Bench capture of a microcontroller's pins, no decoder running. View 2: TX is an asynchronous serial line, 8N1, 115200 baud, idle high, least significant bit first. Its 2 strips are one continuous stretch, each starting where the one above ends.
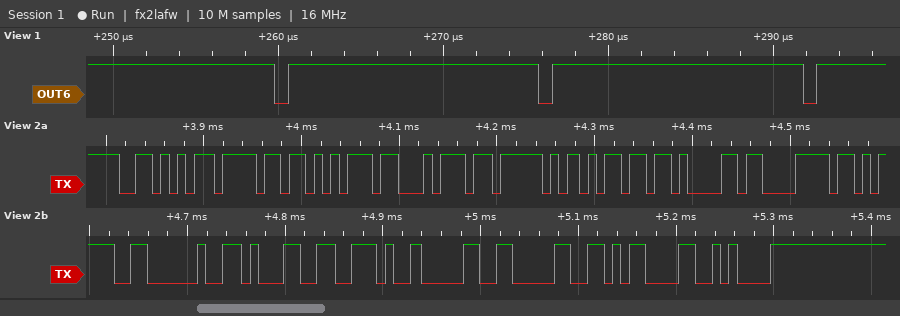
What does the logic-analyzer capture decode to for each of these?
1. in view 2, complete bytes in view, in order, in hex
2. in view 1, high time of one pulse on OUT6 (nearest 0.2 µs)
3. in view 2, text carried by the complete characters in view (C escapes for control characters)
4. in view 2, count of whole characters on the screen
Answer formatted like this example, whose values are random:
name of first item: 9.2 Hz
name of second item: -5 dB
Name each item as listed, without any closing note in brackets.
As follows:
in view 2, complete bytes in view, in order, in hex: 56 6F 75 74 5F 6D 61 78 3D 20 31 2E 30 30 0D 0A
in view 1, high time of one pulse on OUT6: 15.2 µs
in view 2, text carried by the complete characters in view: "Vout_max= 1.00\r\n"
in view 2, count of whole characters on the screen: 16
